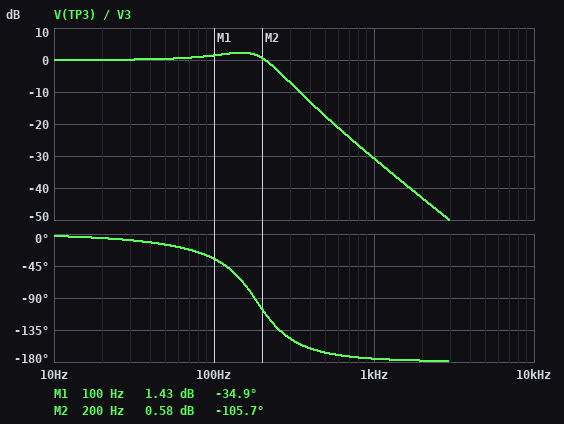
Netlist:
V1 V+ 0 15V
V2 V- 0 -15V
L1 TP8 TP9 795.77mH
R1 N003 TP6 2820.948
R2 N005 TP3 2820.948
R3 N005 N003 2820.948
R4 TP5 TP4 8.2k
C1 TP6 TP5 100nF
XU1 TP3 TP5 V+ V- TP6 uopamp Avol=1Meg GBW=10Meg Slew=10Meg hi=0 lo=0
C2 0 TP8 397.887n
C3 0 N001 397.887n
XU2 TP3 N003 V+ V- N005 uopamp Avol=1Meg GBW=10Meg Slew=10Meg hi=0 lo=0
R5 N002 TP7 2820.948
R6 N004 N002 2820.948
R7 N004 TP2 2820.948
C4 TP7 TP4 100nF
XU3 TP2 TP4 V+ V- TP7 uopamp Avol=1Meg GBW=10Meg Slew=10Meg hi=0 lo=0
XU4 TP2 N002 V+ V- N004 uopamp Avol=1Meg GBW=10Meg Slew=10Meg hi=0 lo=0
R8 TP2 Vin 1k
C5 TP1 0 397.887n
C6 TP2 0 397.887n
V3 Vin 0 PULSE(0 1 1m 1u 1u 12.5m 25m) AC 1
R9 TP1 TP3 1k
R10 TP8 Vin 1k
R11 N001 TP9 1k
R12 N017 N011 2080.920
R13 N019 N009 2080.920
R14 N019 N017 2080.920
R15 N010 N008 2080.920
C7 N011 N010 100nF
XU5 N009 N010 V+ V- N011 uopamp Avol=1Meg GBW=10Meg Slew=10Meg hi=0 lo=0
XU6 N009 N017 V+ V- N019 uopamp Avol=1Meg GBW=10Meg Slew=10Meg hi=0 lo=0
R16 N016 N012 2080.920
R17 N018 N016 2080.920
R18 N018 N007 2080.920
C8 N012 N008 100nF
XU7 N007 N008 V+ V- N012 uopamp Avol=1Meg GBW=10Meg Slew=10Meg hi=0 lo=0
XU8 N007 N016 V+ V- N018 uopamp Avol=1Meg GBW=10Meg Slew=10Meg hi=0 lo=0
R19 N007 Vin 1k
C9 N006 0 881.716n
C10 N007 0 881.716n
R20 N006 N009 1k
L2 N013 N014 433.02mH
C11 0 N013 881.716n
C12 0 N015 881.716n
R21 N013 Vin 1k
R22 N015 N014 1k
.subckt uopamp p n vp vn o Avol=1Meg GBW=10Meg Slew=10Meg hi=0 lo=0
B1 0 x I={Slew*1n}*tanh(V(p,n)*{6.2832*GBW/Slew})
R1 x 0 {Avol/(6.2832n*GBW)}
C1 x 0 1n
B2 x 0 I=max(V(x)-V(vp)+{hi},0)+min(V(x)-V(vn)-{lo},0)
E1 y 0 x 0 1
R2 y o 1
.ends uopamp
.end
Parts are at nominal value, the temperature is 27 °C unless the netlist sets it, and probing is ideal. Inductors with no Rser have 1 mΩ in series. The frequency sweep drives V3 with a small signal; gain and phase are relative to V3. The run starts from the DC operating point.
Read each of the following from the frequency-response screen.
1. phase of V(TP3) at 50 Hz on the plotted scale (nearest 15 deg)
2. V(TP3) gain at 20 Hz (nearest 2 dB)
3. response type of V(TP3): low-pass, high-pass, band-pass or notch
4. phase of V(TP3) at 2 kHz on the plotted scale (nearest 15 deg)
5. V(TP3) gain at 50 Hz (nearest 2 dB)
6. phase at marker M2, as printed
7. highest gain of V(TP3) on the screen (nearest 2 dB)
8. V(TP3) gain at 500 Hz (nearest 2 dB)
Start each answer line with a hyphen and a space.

- -15 deg
- 0 dB
- low-pass
- -180 deg
- 0 dB
- -105.7 deg
- 2 dB
- -18 dB
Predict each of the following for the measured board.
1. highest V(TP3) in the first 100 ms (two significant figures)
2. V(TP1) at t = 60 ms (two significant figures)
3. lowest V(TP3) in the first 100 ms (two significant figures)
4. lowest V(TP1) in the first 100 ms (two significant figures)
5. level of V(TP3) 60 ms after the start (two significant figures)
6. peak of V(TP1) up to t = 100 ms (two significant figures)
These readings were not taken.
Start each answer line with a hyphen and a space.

- 1.2 V
- 1.0 V
- -230 mV
- -200 mV
- 1.0 V
- 1.2 V
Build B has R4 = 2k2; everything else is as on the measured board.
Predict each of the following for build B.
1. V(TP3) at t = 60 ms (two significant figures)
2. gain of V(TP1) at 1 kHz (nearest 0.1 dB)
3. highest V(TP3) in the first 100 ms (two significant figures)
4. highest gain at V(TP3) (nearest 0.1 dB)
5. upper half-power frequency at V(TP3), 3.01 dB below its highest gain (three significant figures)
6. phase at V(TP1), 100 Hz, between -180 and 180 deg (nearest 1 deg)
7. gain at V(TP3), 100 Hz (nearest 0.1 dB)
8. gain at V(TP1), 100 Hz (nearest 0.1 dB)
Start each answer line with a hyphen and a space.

- 1.0 V
- -27.1 dB
- 1.0 V
- 0 dB
- 363 Hz
- -41 deg
- -0.6 dB
- -0.9 dB
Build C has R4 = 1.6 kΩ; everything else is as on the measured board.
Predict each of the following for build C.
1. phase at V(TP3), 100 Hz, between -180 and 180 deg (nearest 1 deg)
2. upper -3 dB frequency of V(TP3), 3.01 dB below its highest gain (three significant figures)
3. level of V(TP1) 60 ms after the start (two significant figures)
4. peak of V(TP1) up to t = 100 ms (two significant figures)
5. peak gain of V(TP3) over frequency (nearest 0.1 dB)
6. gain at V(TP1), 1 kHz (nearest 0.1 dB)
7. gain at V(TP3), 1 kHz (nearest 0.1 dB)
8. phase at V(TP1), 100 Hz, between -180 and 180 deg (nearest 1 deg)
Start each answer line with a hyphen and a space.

- -26 deg
- 290 Hz
- 1.0 V
- 1.0 V
- 0 dB
- -24.1 dB
- -15.5 dB
- -40 deg
